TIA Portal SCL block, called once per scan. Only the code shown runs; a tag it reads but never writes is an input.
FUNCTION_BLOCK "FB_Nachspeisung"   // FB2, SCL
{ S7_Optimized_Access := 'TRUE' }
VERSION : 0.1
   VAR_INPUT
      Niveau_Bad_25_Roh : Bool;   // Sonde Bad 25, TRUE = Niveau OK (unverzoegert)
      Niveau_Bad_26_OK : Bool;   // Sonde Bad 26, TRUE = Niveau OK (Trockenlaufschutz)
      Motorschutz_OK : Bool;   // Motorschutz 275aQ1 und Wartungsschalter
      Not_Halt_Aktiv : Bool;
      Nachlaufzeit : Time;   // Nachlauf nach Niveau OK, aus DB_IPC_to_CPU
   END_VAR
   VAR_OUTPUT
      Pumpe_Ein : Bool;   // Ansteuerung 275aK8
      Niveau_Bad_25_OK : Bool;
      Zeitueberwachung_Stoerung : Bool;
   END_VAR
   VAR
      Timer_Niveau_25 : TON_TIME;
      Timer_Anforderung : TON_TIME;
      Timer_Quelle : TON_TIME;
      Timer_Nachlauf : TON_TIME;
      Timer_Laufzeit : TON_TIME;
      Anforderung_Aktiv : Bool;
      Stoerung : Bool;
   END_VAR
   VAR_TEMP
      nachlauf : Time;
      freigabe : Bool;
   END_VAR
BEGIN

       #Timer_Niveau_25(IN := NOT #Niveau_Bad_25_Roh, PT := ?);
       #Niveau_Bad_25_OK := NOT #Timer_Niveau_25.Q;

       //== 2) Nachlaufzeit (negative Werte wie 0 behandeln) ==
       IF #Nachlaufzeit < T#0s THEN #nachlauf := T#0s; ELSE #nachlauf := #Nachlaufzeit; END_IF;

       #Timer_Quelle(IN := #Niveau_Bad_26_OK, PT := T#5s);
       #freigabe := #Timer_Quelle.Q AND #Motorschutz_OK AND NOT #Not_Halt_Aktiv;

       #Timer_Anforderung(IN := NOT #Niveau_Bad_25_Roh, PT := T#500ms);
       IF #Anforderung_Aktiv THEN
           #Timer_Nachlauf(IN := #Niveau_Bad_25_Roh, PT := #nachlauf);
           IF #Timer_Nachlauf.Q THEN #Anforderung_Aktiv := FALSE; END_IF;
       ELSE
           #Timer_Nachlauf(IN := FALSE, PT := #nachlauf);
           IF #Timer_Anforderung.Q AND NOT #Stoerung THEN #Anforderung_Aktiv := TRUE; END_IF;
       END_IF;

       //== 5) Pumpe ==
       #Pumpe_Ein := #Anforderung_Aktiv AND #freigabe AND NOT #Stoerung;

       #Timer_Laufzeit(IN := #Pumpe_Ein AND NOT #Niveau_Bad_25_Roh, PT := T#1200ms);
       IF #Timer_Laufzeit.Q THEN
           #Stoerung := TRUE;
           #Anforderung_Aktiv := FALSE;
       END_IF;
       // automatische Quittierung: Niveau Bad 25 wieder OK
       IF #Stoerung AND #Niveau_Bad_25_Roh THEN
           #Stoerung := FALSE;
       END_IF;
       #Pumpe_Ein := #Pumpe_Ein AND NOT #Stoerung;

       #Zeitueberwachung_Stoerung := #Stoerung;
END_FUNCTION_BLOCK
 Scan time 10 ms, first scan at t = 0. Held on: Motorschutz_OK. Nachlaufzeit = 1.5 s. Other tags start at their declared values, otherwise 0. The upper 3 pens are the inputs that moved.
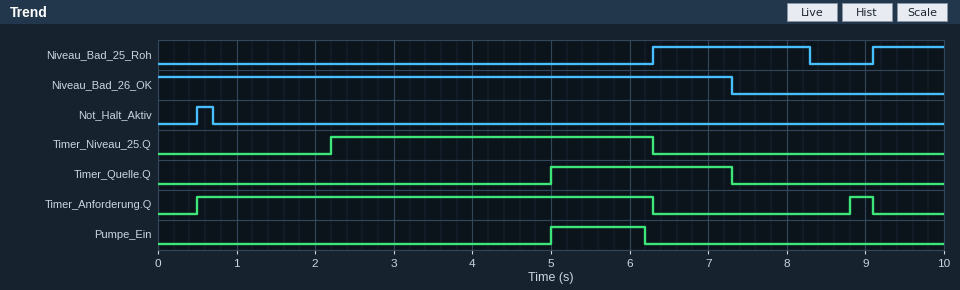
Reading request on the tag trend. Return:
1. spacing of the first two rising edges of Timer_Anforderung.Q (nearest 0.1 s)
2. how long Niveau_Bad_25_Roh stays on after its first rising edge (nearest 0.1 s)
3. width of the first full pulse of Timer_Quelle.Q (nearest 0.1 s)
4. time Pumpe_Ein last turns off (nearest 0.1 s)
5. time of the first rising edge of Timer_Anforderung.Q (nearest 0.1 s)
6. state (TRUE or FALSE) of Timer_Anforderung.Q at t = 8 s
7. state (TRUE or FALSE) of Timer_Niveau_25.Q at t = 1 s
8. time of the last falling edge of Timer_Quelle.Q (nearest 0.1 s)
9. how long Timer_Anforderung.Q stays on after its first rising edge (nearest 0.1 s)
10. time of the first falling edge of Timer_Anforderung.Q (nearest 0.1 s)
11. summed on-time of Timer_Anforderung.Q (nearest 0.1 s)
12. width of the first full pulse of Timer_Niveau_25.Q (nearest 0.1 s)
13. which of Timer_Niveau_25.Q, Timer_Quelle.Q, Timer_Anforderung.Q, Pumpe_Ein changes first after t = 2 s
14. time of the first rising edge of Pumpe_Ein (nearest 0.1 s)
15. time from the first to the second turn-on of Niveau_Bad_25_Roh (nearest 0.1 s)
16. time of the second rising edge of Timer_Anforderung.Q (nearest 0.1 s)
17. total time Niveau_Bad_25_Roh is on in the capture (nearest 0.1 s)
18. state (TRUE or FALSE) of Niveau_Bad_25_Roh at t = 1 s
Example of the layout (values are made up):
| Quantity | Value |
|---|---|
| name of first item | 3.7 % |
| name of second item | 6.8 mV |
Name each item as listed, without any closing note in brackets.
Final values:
| Quantity | Value |
|---|---|
| spacing of the first two rising edges of Timer_Anforderung.Q | 8.3 s |
| how long Niveau_Bad_25_Roh stays on after its first rising edge | 2.0 s |
| width of the first full pulse of Timer_Quelle.Q | 2.3 s |
| time Pumpe_Ein last turns off | 6.2 s |
| time of the first rising edge of Timer_Anforderung.Q | 0.5 s |
| state (TRUE or FALSE) of Timer_Anforderung.Q at t = 8 s | FALSE |
| state (TRUE or FALSE) of Timer_Niveau_25.Q at t = 1 s | FALSE |
| time of the last falling edge of Timer_Quelle.Q | 7.3 s |
| how long Timer_Anforderung.Q stays on after its first rising edge | 5.8 s |
| time of the first falling edge of Timer_Anforderung.Q | 6.3 s |
| summed on-time of Timer_Anforderung.Q | 6.1 s |
| width of the first full pulse of Timer_Niveau_25.Q | 4.1 s |
| which of Timer_Niveau_25.Q, Timer_Quelle.Q, Timer_Anforderung.Q, Pumpe_Ein changes first after t = 2 s | Timer_Niveau_25.Q |
| time of the first rising edge of Pumpe_Ein | 5.0 s |
| time from the first to the second turn-on of Niveau_Bad_25_Roh | 2.8 s |
| time of the second rising edge of Timer_Anforderung.Q | 8.8 s |
| total time Niveau_Bad_25_Roh is on in the capture | 2.9 s |
| state (TRUE or FALSE) of Niveau_Bad_25_Roh at t = 1 s | FALSE |
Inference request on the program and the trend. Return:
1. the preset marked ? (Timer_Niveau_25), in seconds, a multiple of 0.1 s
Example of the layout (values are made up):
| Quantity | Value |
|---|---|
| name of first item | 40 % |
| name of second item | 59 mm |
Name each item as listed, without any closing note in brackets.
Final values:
| Quantity | Value |
|---|---|
| the preset marked ? (Timer_Niveau_25), in seconds, a multiple of 0.1 s | 2.2 s |
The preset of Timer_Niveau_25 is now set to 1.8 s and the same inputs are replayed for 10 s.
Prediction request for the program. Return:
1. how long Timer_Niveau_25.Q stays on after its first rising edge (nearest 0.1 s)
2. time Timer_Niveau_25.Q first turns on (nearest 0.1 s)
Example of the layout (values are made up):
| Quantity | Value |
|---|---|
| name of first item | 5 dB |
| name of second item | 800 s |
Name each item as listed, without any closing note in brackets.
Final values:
| Quantity | Value |
|---|---|
| how long Timer_Niveau_25.Q stays on after its first rising edge | 4.5 s |
| time Timer_Niveau_25.Q first turns on | 1.8 s |
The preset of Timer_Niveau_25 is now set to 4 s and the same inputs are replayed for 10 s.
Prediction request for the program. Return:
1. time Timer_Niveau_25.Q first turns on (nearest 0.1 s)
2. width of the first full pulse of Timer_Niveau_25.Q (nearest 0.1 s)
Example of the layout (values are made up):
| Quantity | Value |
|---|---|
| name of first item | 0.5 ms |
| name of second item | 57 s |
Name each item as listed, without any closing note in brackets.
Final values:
| Quantity | Value |
|---|---|
| time Timer_Niveau_25.Q first turns on | 4.0 s |
| width of the first full pulse of Timer_Niveau_25.Q | 2.3 s |
